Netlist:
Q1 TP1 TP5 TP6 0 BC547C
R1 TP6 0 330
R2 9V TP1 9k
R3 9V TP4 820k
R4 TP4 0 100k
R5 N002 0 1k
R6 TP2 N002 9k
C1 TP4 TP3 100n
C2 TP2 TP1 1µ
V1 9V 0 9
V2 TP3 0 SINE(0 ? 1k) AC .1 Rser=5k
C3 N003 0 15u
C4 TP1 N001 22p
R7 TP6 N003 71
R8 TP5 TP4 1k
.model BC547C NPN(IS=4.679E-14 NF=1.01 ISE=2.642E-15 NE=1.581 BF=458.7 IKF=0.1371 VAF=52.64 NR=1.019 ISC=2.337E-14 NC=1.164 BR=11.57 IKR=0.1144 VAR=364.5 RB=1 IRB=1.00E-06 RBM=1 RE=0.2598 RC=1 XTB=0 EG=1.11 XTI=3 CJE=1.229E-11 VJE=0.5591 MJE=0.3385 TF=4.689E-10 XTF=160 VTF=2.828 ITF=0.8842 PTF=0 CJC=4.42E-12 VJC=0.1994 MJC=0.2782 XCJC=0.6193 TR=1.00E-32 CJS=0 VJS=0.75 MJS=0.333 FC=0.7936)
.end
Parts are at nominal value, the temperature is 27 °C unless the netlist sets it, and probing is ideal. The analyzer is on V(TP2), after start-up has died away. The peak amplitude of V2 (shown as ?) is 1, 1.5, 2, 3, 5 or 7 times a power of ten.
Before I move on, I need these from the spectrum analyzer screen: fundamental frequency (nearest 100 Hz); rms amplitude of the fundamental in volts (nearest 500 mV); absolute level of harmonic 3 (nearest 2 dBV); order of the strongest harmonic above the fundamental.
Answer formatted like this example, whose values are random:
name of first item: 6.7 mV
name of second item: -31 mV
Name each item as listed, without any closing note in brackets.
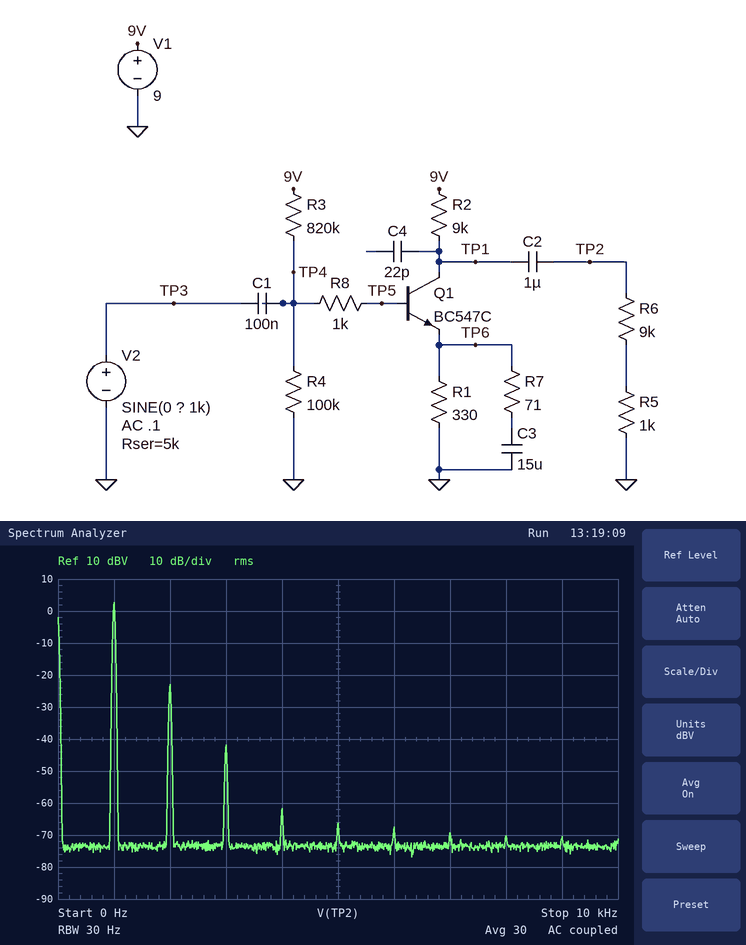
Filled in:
fundamental frequency: 1.0 kHz
rms amplitude of the fundamental in volts: 1.5 V
absolute level of harmonic 3: -42 dBV
order of the strongest harmonic above the fundamental: 2
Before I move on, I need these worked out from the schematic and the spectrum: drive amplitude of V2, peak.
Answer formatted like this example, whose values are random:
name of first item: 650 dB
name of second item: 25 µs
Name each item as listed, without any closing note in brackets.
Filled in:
drive amplitude of V2, peak: 50 mV
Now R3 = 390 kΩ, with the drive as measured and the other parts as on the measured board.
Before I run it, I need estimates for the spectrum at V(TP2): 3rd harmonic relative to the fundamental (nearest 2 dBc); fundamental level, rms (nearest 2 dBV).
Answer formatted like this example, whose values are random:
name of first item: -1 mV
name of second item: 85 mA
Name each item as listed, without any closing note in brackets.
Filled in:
3rd harmonic relative to the fundamental: -20 dBc
fundamental level, rms: -34 dBV
